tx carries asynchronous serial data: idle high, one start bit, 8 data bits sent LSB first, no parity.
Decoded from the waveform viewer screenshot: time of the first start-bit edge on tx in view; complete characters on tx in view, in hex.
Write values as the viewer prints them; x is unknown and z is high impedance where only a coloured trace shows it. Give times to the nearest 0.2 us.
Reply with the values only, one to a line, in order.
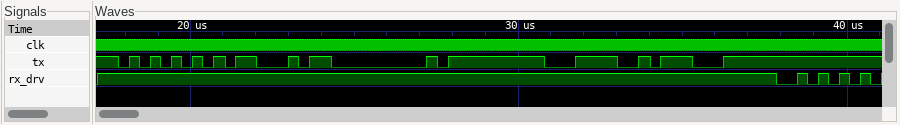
17.8 us
55, A3, 00, FF, 3C, C7
